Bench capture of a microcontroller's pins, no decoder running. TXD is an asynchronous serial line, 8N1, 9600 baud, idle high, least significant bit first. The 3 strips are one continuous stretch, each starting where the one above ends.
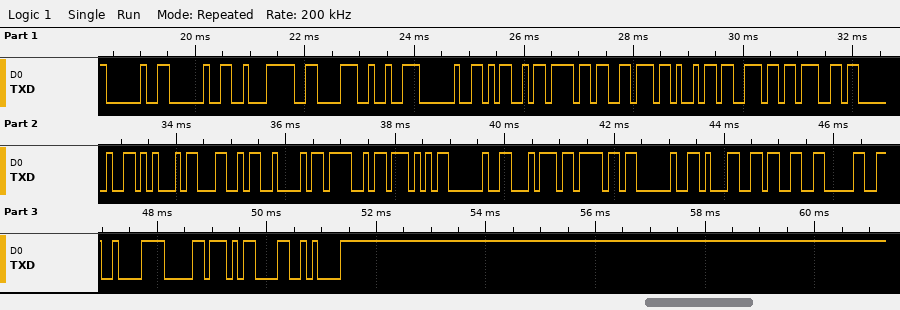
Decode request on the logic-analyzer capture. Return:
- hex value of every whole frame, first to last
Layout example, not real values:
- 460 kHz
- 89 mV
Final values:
- 20 20 E2 86 92 20 4D 6F 76 69 6E 67 20 45 4C 42 4F 57 20 74 6F 20 31 33 30 C2 B0 0D 0A
